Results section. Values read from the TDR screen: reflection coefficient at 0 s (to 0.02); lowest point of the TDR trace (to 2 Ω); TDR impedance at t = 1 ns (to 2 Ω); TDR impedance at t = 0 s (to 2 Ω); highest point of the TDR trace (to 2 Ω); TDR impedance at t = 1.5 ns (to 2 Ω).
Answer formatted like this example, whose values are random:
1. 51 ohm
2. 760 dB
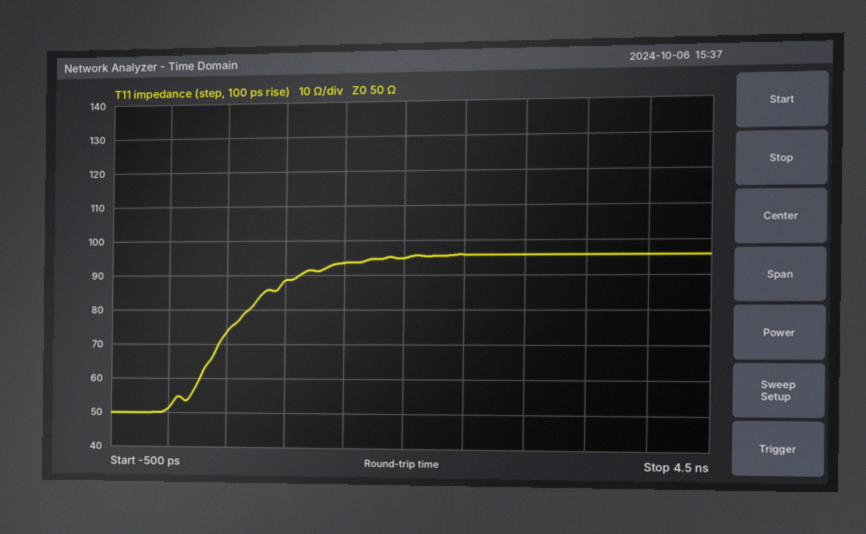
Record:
1. +0.02
2. 50 Ω
3. 88 Ω
4. 52 Ω
5. 96 Ω
6. 94 Ω
